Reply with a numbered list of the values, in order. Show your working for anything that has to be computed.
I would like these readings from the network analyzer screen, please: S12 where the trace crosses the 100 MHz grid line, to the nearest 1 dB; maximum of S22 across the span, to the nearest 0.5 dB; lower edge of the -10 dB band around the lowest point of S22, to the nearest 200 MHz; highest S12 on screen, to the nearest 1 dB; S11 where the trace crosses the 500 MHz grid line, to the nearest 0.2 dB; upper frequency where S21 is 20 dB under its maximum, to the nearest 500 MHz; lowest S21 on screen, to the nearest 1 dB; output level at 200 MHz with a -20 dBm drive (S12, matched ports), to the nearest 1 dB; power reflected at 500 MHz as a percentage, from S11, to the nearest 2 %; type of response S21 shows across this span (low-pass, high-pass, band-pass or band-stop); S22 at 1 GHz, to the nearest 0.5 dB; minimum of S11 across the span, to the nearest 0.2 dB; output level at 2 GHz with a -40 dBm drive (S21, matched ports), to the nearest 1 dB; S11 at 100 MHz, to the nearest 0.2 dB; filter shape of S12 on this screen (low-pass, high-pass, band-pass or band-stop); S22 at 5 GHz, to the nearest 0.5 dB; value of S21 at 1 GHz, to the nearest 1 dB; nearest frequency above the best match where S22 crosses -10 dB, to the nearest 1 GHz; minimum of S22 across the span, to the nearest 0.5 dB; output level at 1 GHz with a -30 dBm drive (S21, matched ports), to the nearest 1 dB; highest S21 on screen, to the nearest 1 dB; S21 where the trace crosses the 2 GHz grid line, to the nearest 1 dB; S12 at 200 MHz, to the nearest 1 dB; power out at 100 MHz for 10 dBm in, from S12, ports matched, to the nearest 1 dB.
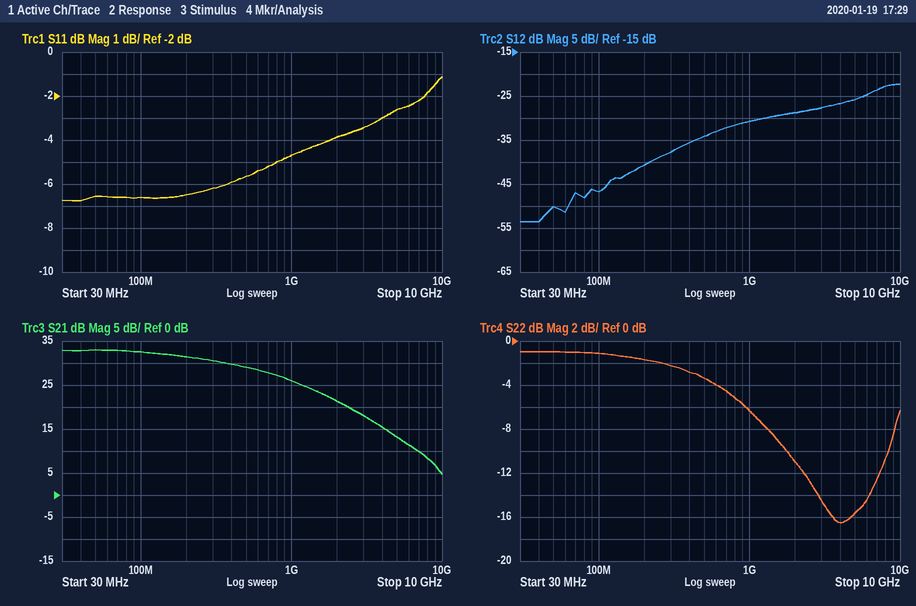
1. -47 dB
2. -1.0 dB
3. 1.8 GHz
4. -22 dB
5. -5.6 dB
6. 5.0 GHz
7. 5 dB
8. -20 dBm + (-41 dB) = -61 dBm
9. 10^(-5.6/10) ≈ 28 %
10. low-pass
11. -6.5 dB
12. -6.8 dB
13. -40 dBm + (21 dB) = -19 dBm
14. -6.6 dB
15. high-pass
16. -15.5 dB
17. 26 dB
18. 8 GHz
19. -16.5 dB
20. -30 dBm + (26 dB) = -4 dBm
21. 33 dB
22. 21 dB
23. -41 dB
24. 10 dBm + (-47 dB) = -37 dBm
